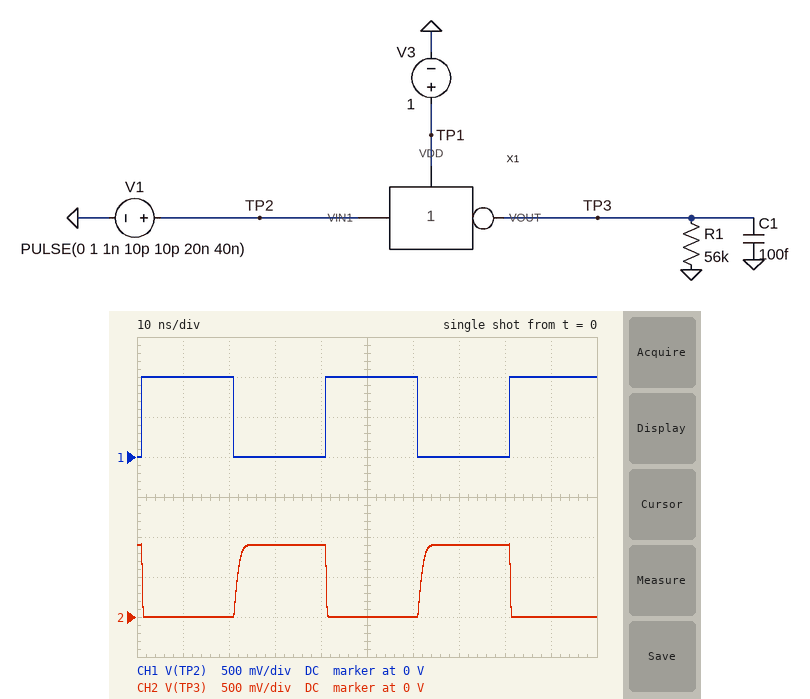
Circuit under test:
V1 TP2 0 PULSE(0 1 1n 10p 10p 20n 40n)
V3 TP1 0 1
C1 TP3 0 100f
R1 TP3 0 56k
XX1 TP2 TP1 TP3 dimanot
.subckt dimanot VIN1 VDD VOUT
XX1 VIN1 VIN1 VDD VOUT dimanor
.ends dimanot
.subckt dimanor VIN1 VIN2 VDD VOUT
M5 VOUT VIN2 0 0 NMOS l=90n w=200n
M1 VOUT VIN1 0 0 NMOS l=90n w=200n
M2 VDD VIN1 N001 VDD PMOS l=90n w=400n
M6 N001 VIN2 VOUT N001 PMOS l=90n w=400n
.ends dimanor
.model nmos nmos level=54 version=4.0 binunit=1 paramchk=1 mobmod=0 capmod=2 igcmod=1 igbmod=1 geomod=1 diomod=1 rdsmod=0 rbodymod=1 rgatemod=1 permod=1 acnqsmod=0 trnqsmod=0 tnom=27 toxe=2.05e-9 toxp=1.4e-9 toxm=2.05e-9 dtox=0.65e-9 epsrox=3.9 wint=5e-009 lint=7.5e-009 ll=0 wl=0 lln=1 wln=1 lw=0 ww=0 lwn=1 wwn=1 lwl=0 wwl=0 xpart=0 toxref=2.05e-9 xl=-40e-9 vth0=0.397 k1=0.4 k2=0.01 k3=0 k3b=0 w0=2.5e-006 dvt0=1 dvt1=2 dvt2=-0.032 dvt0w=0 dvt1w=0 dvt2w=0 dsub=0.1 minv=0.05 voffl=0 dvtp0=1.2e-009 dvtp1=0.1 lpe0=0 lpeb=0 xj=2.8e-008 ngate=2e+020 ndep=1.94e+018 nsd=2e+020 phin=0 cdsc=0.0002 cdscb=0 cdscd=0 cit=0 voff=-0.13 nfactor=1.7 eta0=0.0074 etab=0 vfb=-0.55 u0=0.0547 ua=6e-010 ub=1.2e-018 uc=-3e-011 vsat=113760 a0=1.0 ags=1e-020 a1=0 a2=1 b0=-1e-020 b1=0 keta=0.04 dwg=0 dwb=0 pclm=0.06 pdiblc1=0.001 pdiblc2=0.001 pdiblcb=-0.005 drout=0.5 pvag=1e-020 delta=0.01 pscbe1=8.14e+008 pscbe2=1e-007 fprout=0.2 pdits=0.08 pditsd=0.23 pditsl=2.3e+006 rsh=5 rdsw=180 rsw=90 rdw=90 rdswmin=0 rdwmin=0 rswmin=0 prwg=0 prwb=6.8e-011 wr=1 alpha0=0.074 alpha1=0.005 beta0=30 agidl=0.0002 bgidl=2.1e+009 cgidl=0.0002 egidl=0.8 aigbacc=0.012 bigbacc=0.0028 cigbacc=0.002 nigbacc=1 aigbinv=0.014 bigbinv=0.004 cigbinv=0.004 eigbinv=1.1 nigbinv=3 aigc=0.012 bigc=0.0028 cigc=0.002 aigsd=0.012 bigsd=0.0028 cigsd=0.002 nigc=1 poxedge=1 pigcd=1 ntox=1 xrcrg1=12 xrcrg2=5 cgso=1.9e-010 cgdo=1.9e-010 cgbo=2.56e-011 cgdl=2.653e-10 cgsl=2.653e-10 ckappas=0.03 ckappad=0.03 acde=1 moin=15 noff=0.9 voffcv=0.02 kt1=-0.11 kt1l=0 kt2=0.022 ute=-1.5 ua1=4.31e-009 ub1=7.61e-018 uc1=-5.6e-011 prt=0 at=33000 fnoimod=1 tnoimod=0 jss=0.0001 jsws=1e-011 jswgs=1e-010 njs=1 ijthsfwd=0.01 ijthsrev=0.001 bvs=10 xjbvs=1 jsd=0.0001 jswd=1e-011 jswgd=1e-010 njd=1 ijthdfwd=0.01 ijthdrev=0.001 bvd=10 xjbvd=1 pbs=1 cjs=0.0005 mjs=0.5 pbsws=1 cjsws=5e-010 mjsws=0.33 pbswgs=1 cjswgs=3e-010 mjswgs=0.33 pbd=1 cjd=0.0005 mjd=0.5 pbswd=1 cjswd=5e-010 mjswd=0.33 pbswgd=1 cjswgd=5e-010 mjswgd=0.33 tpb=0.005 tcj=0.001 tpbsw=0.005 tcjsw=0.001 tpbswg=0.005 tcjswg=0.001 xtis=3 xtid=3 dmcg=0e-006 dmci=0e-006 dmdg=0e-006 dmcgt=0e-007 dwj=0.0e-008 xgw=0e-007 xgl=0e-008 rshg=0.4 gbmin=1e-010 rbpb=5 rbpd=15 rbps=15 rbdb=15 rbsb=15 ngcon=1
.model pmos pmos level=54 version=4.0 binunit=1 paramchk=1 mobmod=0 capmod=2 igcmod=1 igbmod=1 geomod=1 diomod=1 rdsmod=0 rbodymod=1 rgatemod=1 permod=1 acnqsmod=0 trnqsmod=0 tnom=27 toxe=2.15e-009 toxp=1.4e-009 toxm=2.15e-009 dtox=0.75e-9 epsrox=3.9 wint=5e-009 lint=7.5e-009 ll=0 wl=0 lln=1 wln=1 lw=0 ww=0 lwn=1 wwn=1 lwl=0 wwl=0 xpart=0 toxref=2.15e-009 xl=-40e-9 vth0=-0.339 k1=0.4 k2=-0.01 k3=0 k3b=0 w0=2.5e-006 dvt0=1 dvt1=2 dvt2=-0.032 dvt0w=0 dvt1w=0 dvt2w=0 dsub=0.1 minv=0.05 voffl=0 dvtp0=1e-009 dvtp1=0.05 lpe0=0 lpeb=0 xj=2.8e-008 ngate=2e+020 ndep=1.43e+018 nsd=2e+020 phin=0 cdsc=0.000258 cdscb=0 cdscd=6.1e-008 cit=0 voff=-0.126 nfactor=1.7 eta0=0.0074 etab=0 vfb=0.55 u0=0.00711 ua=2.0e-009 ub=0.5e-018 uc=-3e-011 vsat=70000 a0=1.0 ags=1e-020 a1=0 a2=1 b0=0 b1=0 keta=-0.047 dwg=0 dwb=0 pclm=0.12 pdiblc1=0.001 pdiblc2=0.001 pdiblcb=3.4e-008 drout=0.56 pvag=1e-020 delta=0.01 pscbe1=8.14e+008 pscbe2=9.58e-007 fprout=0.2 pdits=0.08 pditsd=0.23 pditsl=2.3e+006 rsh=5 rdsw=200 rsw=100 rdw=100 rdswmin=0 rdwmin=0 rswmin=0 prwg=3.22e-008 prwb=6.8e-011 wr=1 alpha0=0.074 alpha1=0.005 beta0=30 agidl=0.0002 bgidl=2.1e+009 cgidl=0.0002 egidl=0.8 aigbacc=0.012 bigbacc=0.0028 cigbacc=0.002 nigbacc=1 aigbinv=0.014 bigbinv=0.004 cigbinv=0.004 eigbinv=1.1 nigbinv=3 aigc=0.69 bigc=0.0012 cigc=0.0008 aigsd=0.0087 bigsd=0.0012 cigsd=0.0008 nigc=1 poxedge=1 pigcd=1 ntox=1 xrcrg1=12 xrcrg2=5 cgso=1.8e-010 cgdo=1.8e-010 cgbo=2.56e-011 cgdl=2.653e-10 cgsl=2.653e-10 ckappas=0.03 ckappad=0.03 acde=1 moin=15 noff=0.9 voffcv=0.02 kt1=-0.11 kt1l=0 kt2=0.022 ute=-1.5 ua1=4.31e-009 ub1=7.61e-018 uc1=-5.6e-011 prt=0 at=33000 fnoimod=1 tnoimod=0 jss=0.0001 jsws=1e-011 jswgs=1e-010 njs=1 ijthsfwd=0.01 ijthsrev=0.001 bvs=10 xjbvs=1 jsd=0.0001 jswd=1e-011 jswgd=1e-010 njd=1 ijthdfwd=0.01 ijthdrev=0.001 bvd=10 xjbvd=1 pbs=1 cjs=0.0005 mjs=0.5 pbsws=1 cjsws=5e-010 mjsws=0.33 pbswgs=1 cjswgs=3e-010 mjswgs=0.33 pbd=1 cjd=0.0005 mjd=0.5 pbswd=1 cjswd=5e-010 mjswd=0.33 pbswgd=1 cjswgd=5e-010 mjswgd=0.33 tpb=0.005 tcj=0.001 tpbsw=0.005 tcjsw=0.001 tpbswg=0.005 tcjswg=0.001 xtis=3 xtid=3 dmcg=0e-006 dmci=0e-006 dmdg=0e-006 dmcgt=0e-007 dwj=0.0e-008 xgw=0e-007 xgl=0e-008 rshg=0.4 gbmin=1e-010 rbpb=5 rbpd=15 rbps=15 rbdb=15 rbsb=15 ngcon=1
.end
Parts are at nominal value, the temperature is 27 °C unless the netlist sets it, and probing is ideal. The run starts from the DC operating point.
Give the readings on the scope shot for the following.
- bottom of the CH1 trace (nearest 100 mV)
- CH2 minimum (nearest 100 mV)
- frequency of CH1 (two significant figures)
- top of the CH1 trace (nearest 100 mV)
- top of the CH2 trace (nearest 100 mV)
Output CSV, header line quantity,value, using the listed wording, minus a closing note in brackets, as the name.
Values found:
quantity,value
bottom of the CH1 trace,0 V
CH2 minimum,0 V
frequency of CH1,25 MHz
top of the CH1 trace,1.0 V
top of the CH2 trace,900 mV
